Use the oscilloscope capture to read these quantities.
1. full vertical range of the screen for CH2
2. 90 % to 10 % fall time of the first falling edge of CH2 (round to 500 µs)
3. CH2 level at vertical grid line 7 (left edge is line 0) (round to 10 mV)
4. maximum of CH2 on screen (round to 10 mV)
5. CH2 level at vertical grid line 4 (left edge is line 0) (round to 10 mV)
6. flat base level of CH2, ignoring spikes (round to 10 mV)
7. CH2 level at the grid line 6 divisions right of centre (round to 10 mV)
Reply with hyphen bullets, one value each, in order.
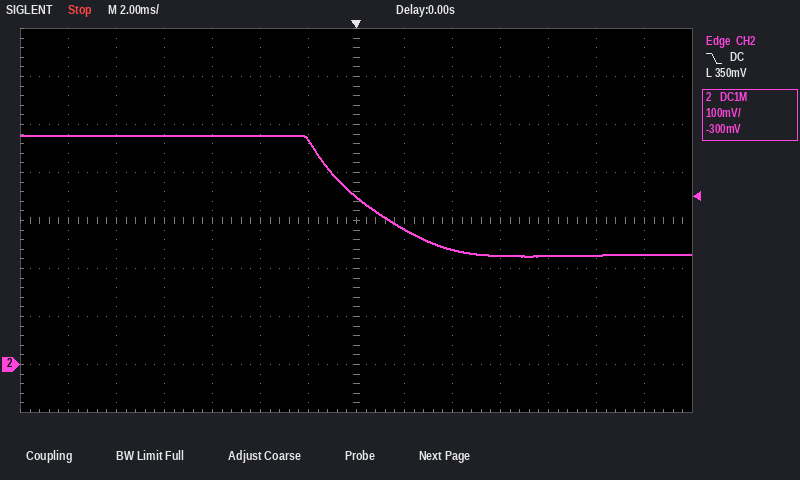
- 800 mV
- 5.0 ms
- 350 mV
- 480 mV
- 480 mV
- 230 mV
- 230 mV
